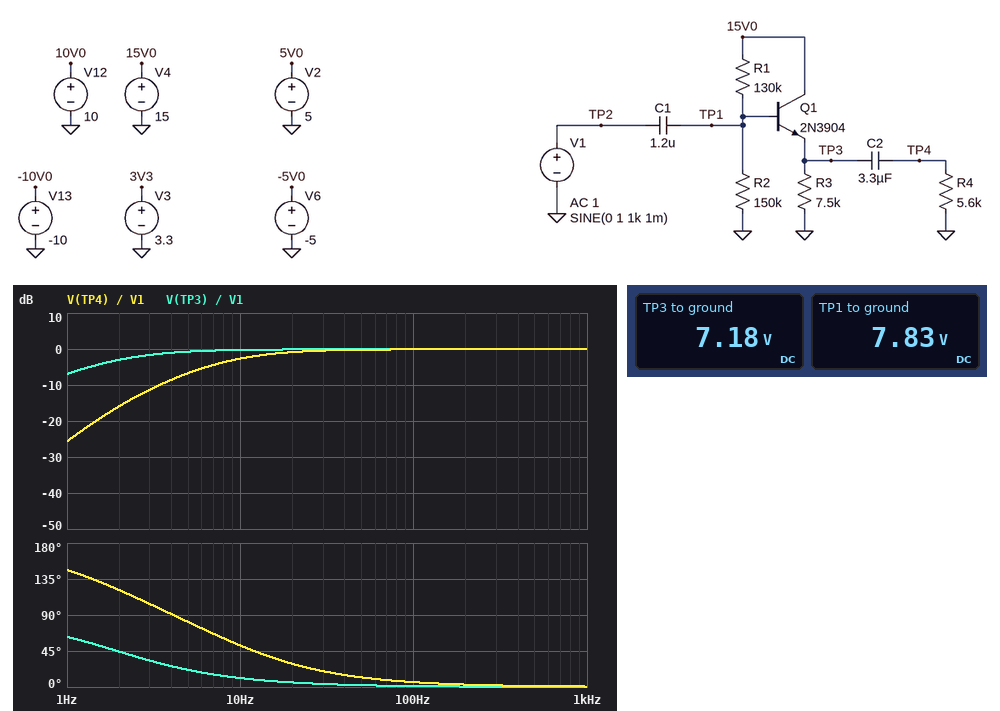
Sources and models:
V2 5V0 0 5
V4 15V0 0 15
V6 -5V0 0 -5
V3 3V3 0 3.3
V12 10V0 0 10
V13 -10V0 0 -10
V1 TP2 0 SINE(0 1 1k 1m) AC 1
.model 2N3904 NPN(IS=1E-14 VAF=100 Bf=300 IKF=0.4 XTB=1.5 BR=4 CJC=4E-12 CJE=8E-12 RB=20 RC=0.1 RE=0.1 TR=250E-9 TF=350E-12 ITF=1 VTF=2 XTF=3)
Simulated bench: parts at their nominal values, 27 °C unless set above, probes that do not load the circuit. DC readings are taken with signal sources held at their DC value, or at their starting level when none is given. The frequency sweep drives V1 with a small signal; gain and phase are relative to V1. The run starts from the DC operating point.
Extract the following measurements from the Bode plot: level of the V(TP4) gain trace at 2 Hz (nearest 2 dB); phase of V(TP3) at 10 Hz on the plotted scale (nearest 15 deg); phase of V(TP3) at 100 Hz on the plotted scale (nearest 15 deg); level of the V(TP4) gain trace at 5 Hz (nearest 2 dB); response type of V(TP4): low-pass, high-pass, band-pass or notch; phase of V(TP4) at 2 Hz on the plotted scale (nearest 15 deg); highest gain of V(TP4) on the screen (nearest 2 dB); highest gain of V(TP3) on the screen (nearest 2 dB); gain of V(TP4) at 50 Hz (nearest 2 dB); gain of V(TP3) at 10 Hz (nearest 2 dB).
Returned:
-16 dB
15 deg
0 deg
-6 dB
high-pass
120 deg
0 dB
0 dB
0 dB
0 dB
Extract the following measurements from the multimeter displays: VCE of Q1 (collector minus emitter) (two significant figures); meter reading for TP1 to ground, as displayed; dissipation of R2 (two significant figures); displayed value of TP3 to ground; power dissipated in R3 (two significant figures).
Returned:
7.8 V
7.83 V
410 µW
7.18 V
6.9 mW
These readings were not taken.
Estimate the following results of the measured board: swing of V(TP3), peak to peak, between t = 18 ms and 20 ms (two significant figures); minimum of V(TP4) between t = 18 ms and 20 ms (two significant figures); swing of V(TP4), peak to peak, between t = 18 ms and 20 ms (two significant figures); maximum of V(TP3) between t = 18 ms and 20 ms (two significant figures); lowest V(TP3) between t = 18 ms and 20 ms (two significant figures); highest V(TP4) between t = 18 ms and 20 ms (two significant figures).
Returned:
2.0 V
-990 mV
2.0 V
8.2 V
6.2 V
990 mV
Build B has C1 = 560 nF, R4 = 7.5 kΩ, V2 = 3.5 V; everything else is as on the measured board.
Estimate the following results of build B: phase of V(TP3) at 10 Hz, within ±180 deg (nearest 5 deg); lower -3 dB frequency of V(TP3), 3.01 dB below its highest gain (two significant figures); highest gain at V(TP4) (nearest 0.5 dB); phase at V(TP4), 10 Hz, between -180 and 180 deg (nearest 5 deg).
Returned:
25 deg
4.3 Hz
0 dB
55 deg
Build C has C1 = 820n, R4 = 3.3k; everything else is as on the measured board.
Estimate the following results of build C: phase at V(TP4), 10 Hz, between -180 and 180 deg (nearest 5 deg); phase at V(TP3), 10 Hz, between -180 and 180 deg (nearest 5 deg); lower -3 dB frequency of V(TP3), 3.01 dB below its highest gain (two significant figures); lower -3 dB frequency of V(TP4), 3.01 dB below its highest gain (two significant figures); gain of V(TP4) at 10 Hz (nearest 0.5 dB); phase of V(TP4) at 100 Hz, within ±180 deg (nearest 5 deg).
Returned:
70 deg
15 deg
2.9 Hz
15 Hz
-5.5 dB
10 deg
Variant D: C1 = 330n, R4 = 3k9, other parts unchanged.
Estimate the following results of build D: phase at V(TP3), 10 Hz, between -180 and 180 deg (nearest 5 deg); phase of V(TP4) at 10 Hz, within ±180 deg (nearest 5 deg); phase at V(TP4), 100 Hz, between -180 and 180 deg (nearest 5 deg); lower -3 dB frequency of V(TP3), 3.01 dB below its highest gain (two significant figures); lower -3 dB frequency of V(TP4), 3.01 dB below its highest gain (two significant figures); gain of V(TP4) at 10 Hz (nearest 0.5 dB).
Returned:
35 deg
85 deg
10 deg
7.3 Hz
16 Hz
-6.0 dB
